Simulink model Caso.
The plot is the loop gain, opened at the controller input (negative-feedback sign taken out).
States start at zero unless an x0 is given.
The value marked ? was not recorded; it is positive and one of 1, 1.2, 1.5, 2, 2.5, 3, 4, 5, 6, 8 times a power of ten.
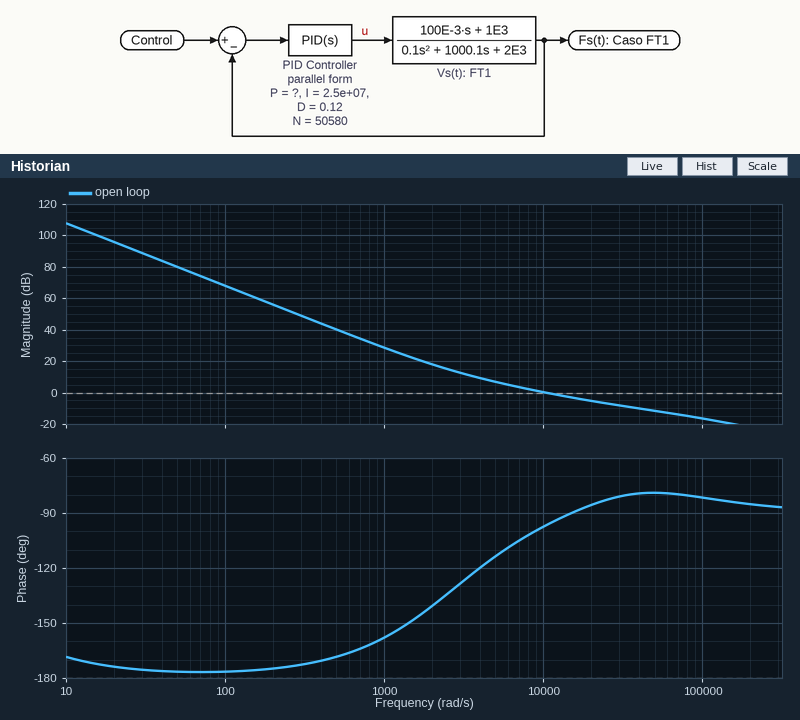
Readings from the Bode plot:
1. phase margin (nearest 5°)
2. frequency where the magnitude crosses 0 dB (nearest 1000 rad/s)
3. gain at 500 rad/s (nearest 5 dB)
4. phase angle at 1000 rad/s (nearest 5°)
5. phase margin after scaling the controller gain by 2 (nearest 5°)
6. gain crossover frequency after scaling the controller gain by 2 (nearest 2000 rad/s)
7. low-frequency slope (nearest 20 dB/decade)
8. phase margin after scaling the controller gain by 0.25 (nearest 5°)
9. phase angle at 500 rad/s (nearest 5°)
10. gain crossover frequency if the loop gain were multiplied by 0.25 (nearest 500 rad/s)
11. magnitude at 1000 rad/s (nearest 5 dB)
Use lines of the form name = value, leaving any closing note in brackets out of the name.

phase margin = 85°
frequency where the magnitude crosses 0 dB = 10000 rad/s
gain at 500 rad/s = 40 dB
phase angle at 1000 rad/s = -160°
phase margin after scaling the controller gain by 2 = 95°
gain crossover frequency after scaling the controller gain by 2 = 22000 rad/s
low-frequency slope = -40 dB/decade
phase margin after scaling the controller gain by 0.25 = 55°
phase angle at 500 rad/s = -170°
gain crossover frequency if the loop gain were multiplied by 0.25 = 3000 rad/s
magnitude at 1000 rad/s = 30 dB
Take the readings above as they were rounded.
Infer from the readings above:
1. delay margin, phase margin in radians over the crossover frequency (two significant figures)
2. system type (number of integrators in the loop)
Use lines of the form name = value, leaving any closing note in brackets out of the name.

delay margin, phase margin in radians over the crossover frequency = 0.00015 s
system type = 2
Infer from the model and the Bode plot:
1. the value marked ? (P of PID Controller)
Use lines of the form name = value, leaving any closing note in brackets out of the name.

the value marked ? = 10000
